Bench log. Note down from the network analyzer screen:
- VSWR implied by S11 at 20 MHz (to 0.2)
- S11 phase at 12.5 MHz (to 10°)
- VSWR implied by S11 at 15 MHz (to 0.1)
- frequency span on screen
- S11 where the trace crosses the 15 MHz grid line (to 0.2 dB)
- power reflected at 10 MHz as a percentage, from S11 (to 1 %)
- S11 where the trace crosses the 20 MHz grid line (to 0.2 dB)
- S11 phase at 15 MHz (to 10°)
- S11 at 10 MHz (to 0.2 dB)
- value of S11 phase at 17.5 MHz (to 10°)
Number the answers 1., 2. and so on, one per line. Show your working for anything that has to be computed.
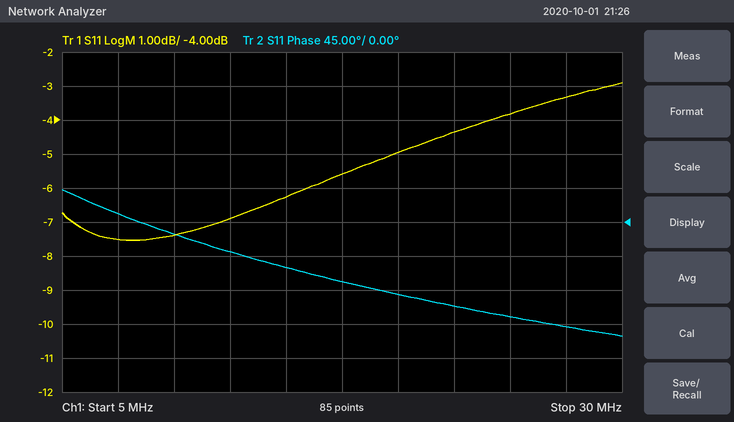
1. |Γ| = 10^(-5/20) = 0.5623; VSWR = (1 + 0.5623)/(1 − 0.5623) ≈ 3.6
2. -40°
3. |Γ| = 10^(-6.2/20) = 0.4898; VSWR = (1 + 0.4898)/(1 − 0.4898) ≈ 2.9
4. 25 MHz
5. -6.2 dB
6. 10^(-7.4/10) ≈ 18 %
7. -5.0 dB
8. -60°
9. -7.4 dB
10. -80°
